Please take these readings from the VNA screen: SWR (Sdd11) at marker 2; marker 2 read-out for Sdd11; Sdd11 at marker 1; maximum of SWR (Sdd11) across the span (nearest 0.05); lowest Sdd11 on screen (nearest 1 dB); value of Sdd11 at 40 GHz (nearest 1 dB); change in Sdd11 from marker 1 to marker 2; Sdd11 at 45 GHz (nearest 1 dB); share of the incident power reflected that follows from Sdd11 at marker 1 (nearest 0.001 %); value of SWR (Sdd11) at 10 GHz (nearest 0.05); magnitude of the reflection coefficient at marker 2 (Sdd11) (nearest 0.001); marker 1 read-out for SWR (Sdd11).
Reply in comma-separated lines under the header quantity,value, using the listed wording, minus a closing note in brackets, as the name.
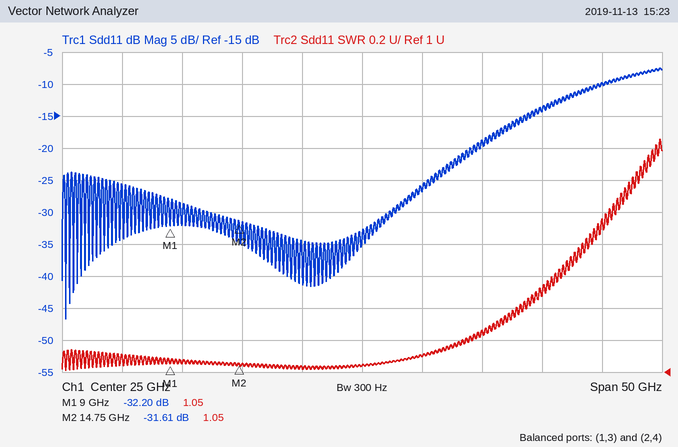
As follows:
quantity,value
SWR (Sdd11) at marker 2,1.05
marker 2 read-out for Sdd11,-31.61 dB
Sdd11 at marker 1,-32.20 dB
maximum of SWR (Sdd11) across the span,2.45
lowest Sdd11 on screen,-47 dB
value of Sdd11 at 40 GHz,-14 dB
change in Sdd11 from marker 1 to marker 2,0.59 dB
Sdd11 at 45 GHz,-10 dB
share of the incident power reflected that follows from Sdd11 at marker 1,0.060 %
value of SWR (Sdd11) at 10 GHz,1.05
magnitude of the reflection coefficient at marker 2 (Sdd11),0.026
marker 1 read-out for SWR,1.05
